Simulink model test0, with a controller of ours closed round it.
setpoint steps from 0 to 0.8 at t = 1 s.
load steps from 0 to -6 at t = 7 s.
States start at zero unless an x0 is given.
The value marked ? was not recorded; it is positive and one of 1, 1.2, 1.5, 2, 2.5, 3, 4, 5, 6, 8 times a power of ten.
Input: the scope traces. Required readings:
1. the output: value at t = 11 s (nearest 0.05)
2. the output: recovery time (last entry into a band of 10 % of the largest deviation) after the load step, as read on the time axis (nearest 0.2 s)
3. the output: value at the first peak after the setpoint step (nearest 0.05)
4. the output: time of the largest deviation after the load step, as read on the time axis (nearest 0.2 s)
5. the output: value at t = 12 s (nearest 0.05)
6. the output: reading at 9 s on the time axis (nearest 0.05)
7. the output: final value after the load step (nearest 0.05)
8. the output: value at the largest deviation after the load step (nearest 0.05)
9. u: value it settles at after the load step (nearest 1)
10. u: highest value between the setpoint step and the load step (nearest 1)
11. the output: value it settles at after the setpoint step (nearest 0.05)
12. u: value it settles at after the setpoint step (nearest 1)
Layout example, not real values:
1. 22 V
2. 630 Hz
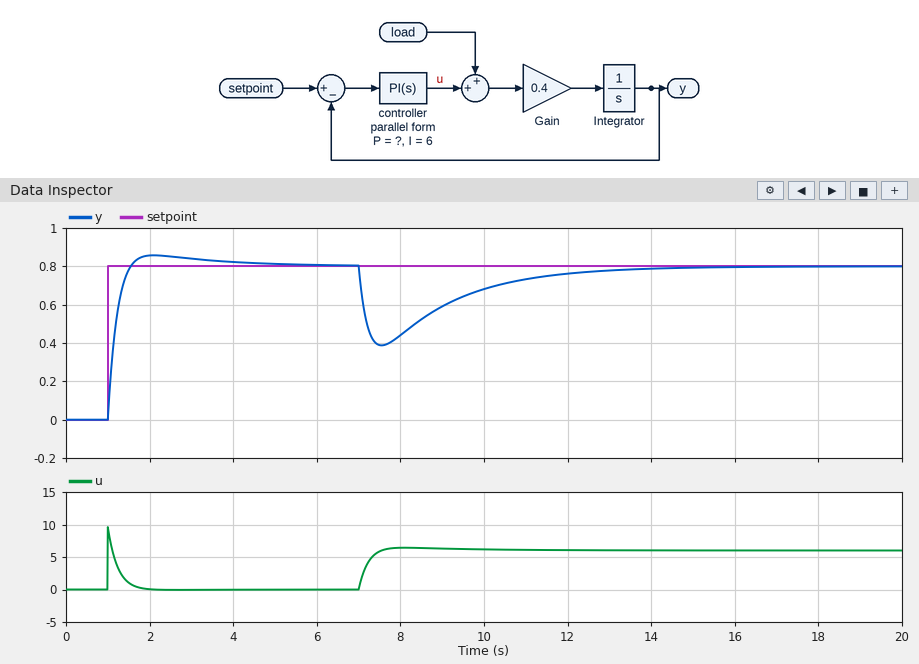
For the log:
1. 0.75
2. 11.8 s
3. 0.85
4. 7.6 s
5. 0.75
6. 0.60
7. 0.80
8. 0.40
9. 6
10. 10
11. 0.80
12. 0
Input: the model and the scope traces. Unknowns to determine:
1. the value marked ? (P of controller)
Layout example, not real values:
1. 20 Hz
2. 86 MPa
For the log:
1. 12
